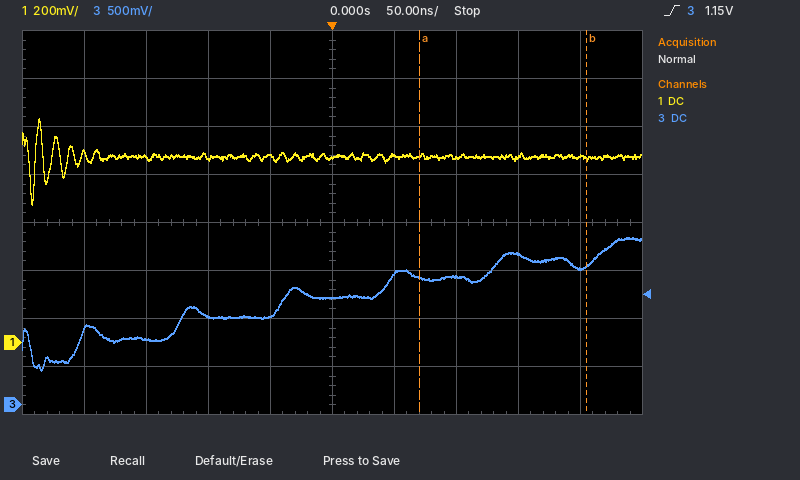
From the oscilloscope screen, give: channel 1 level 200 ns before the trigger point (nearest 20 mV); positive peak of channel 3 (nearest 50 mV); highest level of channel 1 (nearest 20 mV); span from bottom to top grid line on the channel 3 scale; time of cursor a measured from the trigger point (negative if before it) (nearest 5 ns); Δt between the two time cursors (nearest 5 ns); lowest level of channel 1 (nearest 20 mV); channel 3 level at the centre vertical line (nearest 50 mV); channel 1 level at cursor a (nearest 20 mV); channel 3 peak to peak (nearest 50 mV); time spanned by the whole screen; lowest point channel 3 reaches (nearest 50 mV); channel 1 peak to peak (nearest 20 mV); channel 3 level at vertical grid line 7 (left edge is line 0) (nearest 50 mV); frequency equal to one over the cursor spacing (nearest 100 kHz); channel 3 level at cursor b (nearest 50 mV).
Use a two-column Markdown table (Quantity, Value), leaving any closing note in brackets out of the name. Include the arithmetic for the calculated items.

| Quantity | Value |
|---|---|
| channel 1 level 200 ns before the trigger point | 780 mV |
| positive peak of channel 3 | 1.75 V |
| highest level of channel 1 | 940 mV |
| span from bottom to top grid line on the channel 3 scale | 4 V |
| time of cursor a measured from the trigger point (negative if before it) | +70 ns |
| Δt between the two time cursors | 135 ns |
| lowest level of channel 1 | 580 mV |
| channel 3 level at the centre vertical line | 1.10 V |
| channel 1 level at cursor a | 780 mV |
| channel 3 peak to peak | 1.75 V − (350 mV) = 1.40 V |
| time spanned by the whole screen | 500 ns |
| lowest point channel 3 reaches | 350 mV |
| channel 1 peak to peak | 940 mV − (580 mV) = 360 mV |
| channel 3 level at vertical grid line 7 (left edge is line 0) | 1.35 V |
| frequency equal to one over the cursor spacing | 1 / 135 ns ≈ 7.4 MHz |
| channel 3 level at cursor b | 1.45 V |
